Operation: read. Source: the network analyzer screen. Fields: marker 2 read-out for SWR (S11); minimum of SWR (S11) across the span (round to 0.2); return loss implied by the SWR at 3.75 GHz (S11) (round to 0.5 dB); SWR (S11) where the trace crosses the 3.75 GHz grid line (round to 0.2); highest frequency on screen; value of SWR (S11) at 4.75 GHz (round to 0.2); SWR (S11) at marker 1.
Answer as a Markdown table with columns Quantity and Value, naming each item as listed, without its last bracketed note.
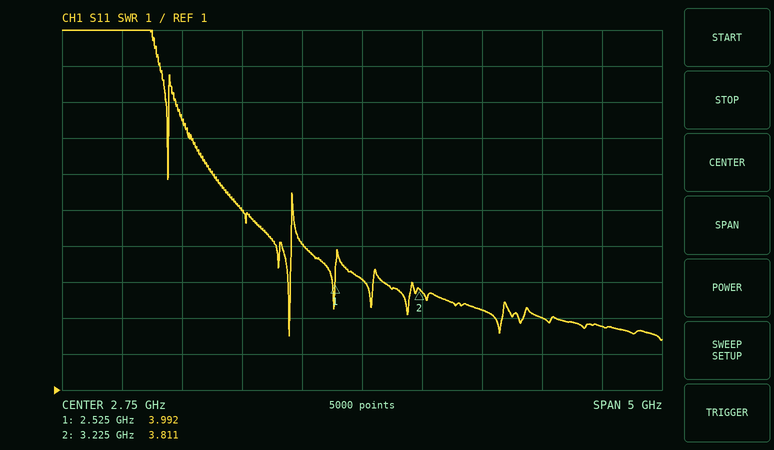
| Quantity | Value |
|---|---|
| marker 2 read-out for SWR | 3.811 |
| minimum of SWR (S11) across the span | 2.4 |
| return loss implied by the SWR at 3.75 GHz (S11) | 5.5 dB |
| SWR (S11) where the trace crosses the 3.75 GHz grid line | 3.2 |
| highest frequency on screen | 5.25 GHz |
| value of SWR (S11) at 4.75 GHz | 2.8 |
| SWR (S11) at marker 1 | 3.992 |
